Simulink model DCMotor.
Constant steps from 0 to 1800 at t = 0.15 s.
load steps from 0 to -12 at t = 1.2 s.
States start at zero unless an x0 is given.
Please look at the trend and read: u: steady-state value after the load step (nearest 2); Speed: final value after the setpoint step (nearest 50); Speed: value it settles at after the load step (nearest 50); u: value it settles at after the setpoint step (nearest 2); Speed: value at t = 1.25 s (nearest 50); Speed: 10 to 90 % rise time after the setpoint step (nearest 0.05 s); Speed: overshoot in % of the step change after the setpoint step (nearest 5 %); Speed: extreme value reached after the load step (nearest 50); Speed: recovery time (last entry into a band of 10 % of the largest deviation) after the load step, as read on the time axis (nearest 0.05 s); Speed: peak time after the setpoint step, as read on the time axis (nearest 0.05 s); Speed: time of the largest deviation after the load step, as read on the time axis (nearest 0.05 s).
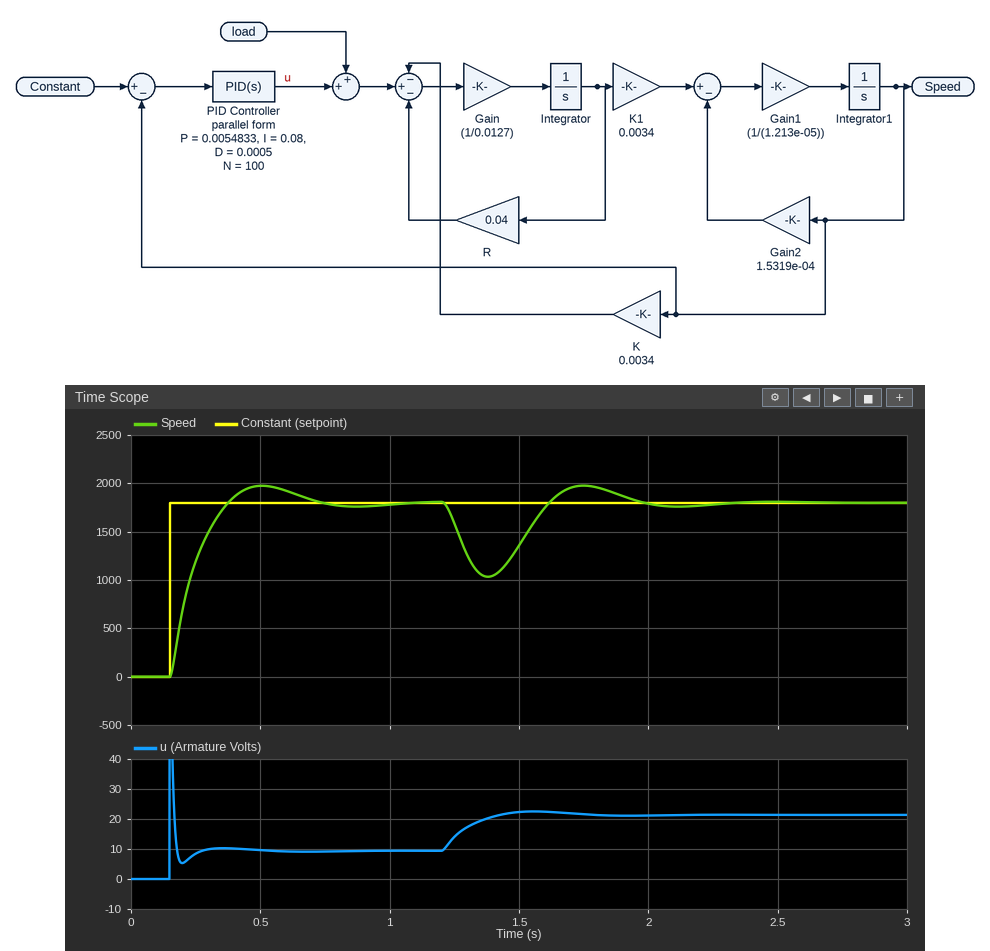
22
1800
1800
10
1600
0.15 s
10 %
1050
1.90 s
0.50 s
1.40 s
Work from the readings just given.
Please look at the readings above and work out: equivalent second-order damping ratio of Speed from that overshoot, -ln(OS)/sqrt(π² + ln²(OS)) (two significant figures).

0.59
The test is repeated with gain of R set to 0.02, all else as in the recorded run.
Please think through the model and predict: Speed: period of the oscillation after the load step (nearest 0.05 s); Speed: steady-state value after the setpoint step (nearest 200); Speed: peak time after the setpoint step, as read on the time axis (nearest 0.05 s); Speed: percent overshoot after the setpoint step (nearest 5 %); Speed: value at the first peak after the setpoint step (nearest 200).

0.70 s
1800
0.45 s
15 %
2000
